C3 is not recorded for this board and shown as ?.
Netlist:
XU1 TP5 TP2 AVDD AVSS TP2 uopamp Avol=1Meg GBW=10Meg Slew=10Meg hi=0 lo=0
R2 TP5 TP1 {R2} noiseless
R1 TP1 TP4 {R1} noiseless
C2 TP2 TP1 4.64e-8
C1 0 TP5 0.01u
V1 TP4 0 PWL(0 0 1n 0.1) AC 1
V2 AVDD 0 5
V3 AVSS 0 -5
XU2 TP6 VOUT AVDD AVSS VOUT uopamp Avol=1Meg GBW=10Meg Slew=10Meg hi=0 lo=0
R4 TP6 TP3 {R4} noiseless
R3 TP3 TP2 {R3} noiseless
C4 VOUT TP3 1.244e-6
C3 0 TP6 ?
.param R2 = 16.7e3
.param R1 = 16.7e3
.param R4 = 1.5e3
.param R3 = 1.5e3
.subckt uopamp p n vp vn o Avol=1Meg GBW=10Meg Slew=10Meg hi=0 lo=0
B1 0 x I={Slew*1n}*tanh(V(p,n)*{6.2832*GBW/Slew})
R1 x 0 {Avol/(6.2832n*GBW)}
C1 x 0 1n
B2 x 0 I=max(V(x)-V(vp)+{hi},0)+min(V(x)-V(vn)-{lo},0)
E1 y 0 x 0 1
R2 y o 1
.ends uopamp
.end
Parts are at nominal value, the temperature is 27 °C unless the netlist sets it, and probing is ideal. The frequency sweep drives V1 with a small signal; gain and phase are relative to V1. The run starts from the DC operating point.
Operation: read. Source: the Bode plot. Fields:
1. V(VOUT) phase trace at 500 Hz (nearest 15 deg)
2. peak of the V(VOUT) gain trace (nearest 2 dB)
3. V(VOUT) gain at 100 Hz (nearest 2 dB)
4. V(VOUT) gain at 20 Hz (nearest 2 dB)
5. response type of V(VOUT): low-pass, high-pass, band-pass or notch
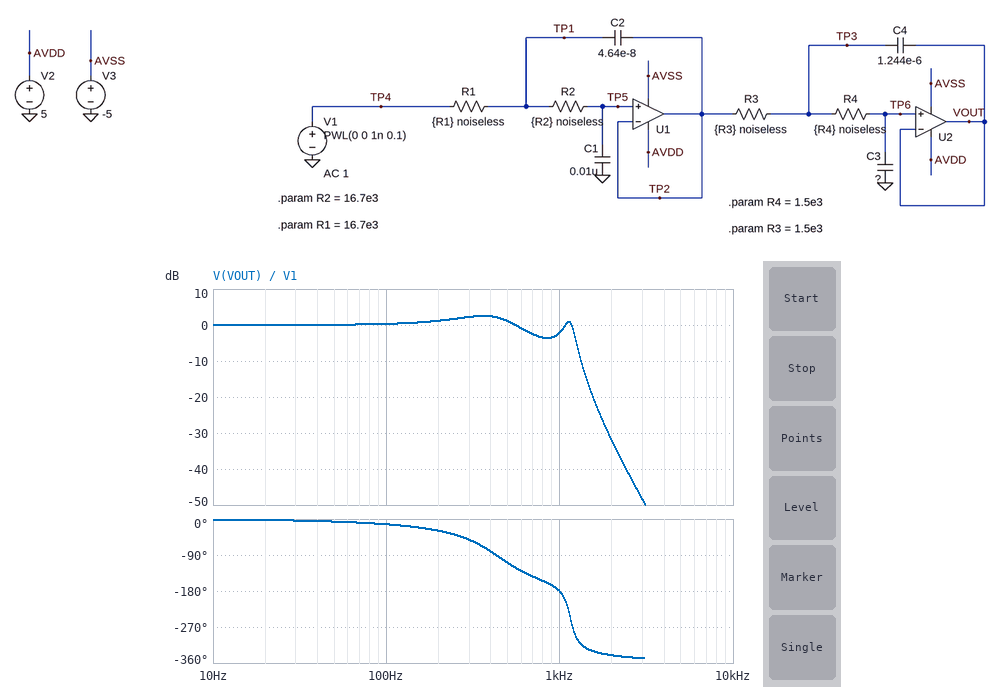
-105 deg
2 dB
0 dB
0 dB
low-pass
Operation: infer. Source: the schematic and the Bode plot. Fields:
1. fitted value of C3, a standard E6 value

6.8 nF
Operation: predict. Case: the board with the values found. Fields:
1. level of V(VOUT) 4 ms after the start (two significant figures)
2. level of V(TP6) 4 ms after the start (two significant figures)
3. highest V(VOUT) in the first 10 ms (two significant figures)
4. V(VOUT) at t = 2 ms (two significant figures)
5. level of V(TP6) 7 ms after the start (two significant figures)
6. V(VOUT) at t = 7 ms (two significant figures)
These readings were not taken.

99 mV
99 mV
120 mV
99 mV
100 mV
100 mV
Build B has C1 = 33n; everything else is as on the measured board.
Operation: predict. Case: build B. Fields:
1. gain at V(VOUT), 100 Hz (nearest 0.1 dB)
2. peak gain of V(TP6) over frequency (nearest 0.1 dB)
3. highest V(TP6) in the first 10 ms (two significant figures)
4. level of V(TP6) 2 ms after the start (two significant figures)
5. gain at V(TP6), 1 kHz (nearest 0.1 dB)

-0.6 dB
0 dB
100 mV
88 mV
-13.7 dB
